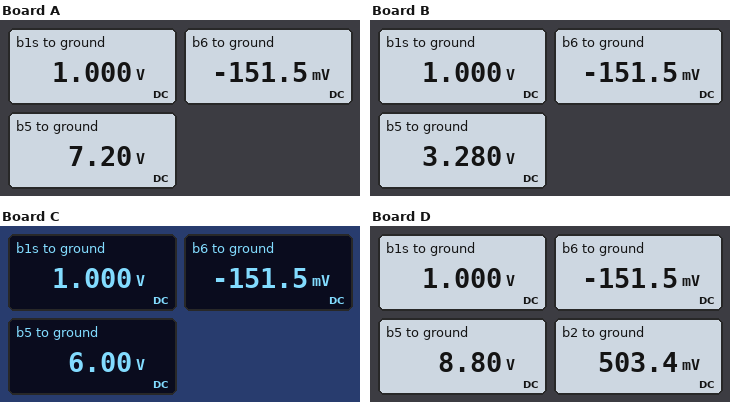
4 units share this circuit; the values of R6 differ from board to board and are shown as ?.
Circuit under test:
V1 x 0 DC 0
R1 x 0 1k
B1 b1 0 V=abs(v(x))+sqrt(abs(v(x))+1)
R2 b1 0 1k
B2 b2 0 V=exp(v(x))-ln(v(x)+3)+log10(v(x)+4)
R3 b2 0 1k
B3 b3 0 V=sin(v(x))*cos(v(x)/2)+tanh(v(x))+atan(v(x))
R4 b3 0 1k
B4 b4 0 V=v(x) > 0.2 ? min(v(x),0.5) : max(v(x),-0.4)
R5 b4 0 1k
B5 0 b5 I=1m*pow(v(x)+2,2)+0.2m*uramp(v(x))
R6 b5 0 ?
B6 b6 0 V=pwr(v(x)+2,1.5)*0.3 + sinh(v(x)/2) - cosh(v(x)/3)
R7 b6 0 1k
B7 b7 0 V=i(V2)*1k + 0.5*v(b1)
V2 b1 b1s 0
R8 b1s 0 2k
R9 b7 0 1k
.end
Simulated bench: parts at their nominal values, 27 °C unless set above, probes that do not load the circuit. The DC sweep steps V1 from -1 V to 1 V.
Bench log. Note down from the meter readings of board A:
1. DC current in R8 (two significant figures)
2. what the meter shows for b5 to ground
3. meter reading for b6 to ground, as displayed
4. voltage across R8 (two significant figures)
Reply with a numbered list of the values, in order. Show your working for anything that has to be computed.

1. (1 V) / 2 kΩ = 500 µA
2. 7.20 V
3. -151.5 mV
4. 1 V = 1.0 V
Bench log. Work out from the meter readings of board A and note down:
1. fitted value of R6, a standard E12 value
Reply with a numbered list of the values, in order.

1. 1.8 kΩ
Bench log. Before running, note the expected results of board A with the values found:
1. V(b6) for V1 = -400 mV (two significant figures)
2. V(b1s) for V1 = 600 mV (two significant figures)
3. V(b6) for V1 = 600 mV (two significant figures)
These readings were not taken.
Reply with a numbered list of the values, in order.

1. -600 mV
2. 1.9 V
3. 540 mV
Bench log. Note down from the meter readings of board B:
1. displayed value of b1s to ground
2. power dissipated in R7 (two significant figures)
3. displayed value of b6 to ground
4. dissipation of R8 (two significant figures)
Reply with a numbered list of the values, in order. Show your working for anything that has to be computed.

1. 1.000 V
2. (0 V - (-151.5 mV))^2 / 1 kΩ = 23 µW
3. -151.5 mV
4. (1 V)^2 / 2 kΩ = 500 µW
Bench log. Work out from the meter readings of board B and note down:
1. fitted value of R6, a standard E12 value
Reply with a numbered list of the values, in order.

1. 820 Ω
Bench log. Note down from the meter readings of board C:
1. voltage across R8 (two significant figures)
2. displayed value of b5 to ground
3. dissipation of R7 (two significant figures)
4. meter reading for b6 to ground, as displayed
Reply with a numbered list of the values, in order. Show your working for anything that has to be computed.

1. 1 V = 1.0 V
2. 6.00 V
3. (0 V - (-151.5 mV))^2 / 1 kΩ = 23 µW
4. -151.5 mV
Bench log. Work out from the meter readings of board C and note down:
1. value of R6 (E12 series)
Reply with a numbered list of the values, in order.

1. 1.5 kΩ
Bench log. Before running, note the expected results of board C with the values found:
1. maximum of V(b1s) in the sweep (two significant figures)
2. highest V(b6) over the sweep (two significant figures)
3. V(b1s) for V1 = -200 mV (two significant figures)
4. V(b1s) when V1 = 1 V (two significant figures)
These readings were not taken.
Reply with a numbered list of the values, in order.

1. 2.4 V
2. 1.0 V
3. 1.3 V
4. 2.4 V
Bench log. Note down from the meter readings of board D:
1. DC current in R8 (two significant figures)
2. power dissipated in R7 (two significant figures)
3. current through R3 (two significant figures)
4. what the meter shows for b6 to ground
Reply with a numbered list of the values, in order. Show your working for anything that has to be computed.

1. (1 V) / 2 kΩ = 500 µA
2. (0 V - (-151.5 mV))^2 / 1 kΩ = 23 µW
3. (503.4 mV) / 1 kΩ = 500 µA
4. -151.5 mV
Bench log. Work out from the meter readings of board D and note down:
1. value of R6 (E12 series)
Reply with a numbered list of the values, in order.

1. 2.2 kΩ
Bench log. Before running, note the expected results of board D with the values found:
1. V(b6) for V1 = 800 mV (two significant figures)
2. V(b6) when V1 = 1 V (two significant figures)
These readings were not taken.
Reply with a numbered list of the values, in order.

1. 780 mV
2. 1.0 V
